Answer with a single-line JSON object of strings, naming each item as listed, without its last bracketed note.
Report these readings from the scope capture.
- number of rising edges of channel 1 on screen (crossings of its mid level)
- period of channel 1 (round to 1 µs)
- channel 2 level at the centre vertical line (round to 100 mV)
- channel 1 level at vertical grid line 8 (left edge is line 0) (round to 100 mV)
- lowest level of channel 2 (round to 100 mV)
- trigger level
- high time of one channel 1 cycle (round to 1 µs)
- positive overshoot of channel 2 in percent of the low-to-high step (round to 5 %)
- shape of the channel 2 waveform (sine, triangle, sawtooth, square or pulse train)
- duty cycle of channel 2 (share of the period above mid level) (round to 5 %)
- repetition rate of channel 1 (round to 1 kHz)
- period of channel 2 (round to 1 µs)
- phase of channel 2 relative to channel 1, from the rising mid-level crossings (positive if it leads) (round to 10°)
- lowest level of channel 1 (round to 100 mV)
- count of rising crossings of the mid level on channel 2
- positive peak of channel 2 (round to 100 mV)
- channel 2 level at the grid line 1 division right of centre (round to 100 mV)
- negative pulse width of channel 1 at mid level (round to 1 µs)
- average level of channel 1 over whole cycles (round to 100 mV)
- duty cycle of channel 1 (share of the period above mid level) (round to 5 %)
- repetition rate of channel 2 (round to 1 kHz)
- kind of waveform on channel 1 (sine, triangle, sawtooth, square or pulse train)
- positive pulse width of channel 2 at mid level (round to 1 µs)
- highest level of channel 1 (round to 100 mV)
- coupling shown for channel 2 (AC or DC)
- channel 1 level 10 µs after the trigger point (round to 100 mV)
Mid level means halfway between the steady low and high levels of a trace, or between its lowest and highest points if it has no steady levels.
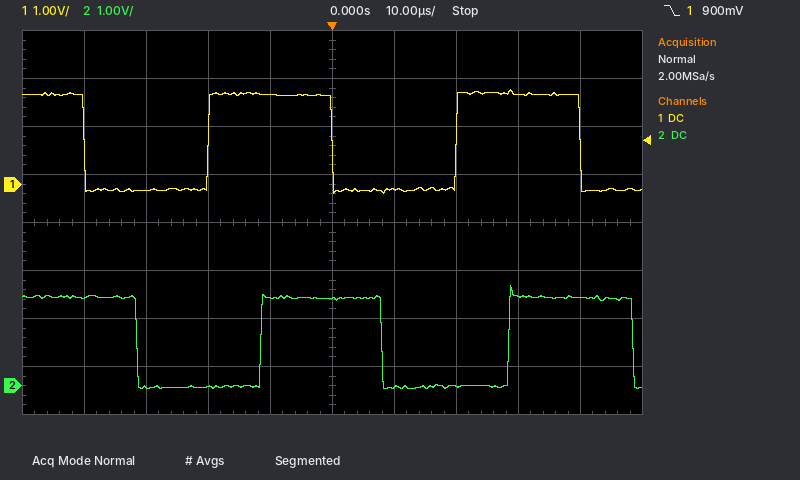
{"number of rising edges of channel 1 on screen": "2", "period of channel 1": "40 µs", "channel 2 level at the centre vertical line": "1.8 V", "channel 1 level at vertical grid line 8 (left edge is line 0)": "1.9 V", "lowest level of channel 2": "-100 mV", "trigger level": "900 mV", "high time of one channel 1 cycle": "20 µs", "positive overshoot of channel 2 in percent of the low-to-high step": "15 %", "shape of the channel 2 waveform": "square", "duty cycle of channel 2 (share of the period above mid level)": "50 %", "repetition rate of channel 1": "25 kHz", "period of channel 2": "40 µs", "phase of channel 2 relative to channel 1, from the rising mid-level crossings (positive if it leads)": "-80°", "lowest level of channel 1": "-200 mV", "count of rising crossings of the mid level on channel 2": "2", "positive peak of channel 2": "2.1 V", "channel 2 level at the grid line 1 division right of centre": "0.0 V", "negative pulse width of channel 1 at mid level": "20 µs", "average level of channel 1 over whole cycles": "900 mV", "duty cycle of channel 1 (share of the period above mid level)": "50 %", "repetition rate of channel 2": "25 kHz", "kind of waveform on channel 1": "square", "positive pulse width of channel 2 at mid level": "20 µs", "highest level of channel 1": "2.0 V", "coupling shown for channel 2": "DC", "channel 1 level 10 µs after the trigger point": "-100 mV"}
